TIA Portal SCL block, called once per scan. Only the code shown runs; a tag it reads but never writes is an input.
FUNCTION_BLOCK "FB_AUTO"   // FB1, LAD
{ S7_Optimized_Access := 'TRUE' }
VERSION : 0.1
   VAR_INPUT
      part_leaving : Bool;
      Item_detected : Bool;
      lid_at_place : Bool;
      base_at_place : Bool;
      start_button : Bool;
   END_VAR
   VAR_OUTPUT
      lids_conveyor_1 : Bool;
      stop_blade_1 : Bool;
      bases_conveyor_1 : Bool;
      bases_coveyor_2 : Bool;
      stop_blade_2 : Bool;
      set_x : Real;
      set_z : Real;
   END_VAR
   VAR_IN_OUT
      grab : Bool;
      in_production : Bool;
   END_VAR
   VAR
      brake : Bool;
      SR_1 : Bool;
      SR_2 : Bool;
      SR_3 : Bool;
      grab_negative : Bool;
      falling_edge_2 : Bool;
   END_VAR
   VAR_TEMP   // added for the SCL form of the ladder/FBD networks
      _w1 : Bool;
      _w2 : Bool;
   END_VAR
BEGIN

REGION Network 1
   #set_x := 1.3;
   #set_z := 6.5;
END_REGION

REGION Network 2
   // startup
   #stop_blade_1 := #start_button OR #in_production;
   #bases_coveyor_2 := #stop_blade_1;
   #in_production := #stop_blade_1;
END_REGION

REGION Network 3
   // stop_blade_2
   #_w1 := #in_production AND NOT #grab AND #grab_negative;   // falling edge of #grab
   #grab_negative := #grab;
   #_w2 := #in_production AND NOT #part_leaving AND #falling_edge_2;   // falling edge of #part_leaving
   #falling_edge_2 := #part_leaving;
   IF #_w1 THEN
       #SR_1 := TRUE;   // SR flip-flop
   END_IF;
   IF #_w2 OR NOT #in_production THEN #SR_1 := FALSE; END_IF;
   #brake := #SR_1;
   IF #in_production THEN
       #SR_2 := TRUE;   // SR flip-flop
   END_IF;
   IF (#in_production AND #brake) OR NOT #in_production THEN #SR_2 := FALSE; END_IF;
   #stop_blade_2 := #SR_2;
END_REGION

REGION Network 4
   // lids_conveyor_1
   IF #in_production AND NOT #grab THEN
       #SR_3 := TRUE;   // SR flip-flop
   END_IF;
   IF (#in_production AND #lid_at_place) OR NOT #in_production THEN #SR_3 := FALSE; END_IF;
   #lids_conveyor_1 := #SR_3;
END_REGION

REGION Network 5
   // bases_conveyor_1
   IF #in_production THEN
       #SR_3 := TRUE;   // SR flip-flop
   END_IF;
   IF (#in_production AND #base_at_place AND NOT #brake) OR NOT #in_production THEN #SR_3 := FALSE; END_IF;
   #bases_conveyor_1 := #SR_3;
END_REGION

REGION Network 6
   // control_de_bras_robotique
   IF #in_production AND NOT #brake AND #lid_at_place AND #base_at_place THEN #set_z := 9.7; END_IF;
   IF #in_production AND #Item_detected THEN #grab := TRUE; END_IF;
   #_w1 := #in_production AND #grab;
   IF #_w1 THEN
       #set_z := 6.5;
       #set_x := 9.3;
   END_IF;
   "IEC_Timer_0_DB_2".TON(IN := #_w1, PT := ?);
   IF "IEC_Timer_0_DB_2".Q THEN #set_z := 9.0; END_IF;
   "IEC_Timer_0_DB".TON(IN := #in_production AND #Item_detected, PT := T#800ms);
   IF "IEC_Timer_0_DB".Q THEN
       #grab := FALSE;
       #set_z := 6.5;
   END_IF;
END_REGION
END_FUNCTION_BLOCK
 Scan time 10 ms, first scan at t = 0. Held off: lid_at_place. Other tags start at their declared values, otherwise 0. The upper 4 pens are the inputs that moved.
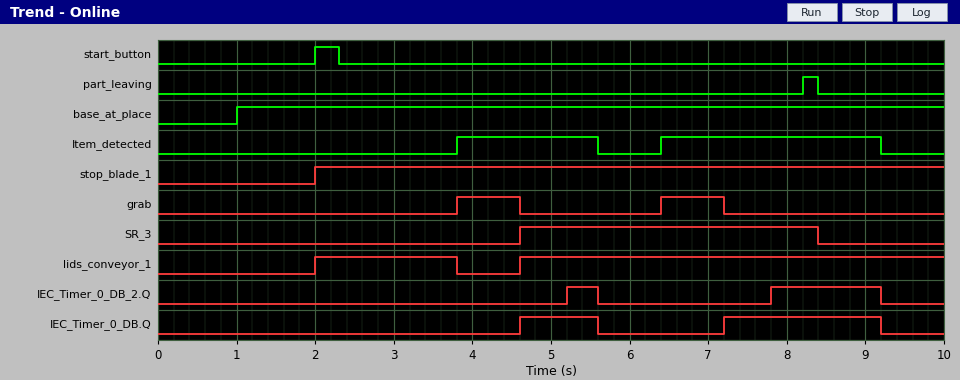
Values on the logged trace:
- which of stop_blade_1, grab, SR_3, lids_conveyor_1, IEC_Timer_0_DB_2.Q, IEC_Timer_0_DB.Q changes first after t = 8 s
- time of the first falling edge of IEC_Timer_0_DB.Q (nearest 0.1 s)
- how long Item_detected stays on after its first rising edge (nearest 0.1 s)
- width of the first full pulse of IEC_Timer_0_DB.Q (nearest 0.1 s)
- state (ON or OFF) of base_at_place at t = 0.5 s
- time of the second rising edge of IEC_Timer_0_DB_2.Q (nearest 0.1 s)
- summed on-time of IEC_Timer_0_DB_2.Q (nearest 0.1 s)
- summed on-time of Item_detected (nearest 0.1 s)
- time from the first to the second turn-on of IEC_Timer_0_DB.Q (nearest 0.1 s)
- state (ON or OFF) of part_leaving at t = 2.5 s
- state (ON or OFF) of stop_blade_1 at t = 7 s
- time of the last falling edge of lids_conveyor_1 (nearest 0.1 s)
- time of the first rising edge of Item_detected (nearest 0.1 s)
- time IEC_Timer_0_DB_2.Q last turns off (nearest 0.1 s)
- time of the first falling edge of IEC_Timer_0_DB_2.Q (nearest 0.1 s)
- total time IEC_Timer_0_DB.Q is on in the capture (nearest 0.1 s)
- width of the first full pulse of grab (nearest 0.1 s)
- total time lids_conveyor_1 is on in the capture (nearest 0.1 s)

SR_3
5.6 s
1.8 s
1.0 s
OFF
7.8 s
1.8 s
4.6 s
2.6 s
OFF
ON
3.8 s
3.8 s
9.2 s
5.6 s
3.0 s
0.8 s
7.2 s
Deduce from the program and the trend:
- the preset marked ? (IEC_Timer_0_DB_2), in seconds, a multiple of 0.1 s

1.4 s
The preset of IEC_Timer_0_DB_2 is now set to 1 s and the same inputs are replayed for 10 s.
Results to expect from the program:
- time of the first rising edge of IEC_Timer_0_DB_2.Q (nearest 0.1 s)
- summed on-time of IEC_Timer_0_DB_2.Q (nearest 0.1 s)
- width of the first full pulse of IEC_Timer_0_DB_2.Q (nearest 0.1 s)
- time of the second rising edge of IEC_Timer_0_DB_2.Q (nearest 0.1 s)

4.8 s
2.6 s
0.8 s
7.4 s
